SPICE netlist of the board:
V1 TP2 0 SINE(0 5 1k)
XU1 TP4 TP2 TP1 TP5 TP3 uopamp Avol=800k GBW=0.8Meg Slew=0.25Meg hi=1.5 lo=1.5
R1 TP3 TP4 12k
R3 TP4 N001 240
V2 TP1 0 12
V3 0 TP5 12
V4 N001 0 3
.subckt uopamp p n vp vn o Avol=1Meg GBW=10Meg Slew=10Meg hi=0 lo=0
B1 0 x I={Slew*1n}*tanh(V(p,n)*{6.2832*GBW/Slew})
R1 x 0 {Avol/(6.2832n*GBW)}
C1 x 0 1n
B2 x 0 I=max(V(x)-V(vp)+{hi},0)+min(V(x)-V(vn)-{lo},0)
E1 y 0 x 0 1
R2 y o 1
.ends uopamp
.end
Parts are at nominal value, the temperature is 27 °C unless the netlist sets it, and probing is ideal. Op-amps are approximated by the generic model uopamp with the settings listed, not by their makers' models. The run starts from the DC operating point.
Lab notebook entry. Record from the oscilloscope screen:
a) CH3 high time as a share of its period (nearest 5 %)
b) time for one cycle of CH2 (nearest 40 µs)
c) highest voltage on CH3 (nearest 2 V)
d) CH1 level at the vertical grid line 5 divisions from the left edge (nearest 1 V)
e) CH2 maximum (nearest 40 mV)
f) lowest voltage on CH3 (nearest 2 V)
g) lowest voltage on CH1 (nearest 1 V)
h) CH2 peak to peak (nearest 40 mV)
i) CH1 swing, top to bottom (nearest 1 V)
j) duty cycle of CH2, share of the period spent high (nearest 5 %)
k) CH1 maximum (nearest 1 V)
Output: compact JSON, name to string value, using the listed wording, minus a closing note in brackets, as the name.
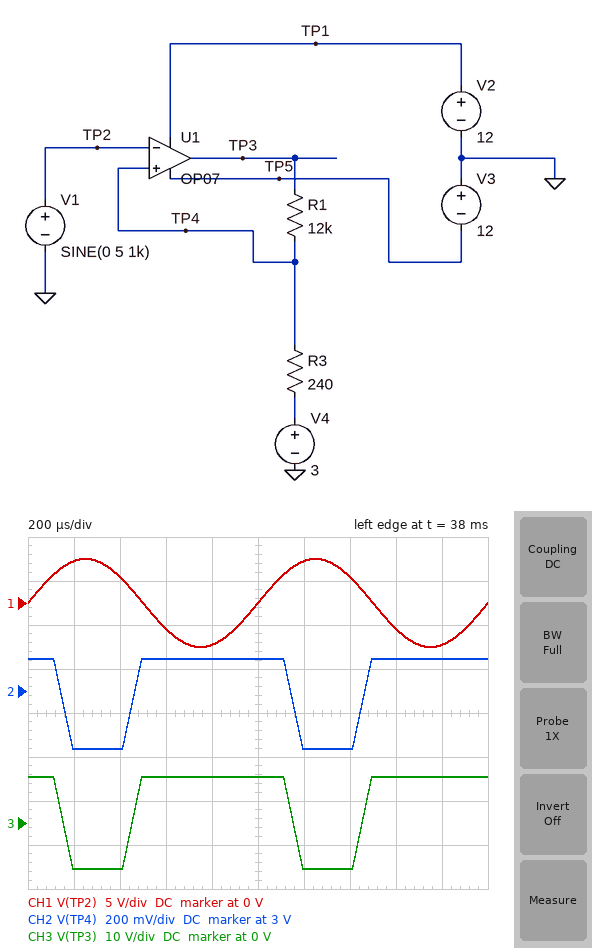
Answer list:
{"CH3 high time as a share of its period": "70 %", "time for one cycle of CH2": "1.00 ms", "highest voltage on CH3": "10 V", "CH1 level at the vertical grid line 5 divisions from the left edge": "0 V", "CH2 maximum": "3.16 V", "lowest voltage on CH3": "-10 V", "lowest voltage on CH1": "-5 V", "CH2 peak to peak": "400 mV", "CH1 swing, top to bottom": "10 V", "duty cycle of CH2, share of the period spent high": "70 %", "CH1 maximum": "5 V"}
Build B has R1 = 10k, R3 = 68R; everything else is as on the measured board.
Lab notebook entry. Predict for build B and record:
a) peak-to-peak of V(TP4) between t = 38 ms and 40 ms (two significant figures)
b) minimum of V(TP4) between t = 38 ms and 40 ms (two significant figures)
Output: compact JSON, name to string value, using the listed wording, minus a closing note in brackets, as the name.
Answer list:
{"peak-to-peak of V(TP4) between t = 38 ms and 40 ms": "140 mV", "minimum of V(TP4) between t = 38 ms and 40 ms": "2.9 V"}
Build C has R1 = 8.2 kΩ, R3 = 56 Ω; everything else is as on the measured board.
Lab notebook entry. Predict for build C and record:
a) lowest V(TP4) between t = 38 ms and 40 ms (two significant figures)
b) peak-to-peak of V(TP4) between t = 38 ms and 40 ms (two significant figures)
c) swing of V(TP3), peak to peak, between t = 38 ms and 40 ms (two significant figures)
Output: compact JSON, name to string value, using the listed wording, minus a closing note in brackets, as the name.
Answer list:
{"lowest V(TP4) between t = 38 ms and 40 ms": "2.9 V", "peak-to-peak of V(TP4) between t = 38 ms and 40 ms": "140 mV", "swing of V(TP3), peak to peak, between t = 38 ms and 40 ms": "21 V"}
